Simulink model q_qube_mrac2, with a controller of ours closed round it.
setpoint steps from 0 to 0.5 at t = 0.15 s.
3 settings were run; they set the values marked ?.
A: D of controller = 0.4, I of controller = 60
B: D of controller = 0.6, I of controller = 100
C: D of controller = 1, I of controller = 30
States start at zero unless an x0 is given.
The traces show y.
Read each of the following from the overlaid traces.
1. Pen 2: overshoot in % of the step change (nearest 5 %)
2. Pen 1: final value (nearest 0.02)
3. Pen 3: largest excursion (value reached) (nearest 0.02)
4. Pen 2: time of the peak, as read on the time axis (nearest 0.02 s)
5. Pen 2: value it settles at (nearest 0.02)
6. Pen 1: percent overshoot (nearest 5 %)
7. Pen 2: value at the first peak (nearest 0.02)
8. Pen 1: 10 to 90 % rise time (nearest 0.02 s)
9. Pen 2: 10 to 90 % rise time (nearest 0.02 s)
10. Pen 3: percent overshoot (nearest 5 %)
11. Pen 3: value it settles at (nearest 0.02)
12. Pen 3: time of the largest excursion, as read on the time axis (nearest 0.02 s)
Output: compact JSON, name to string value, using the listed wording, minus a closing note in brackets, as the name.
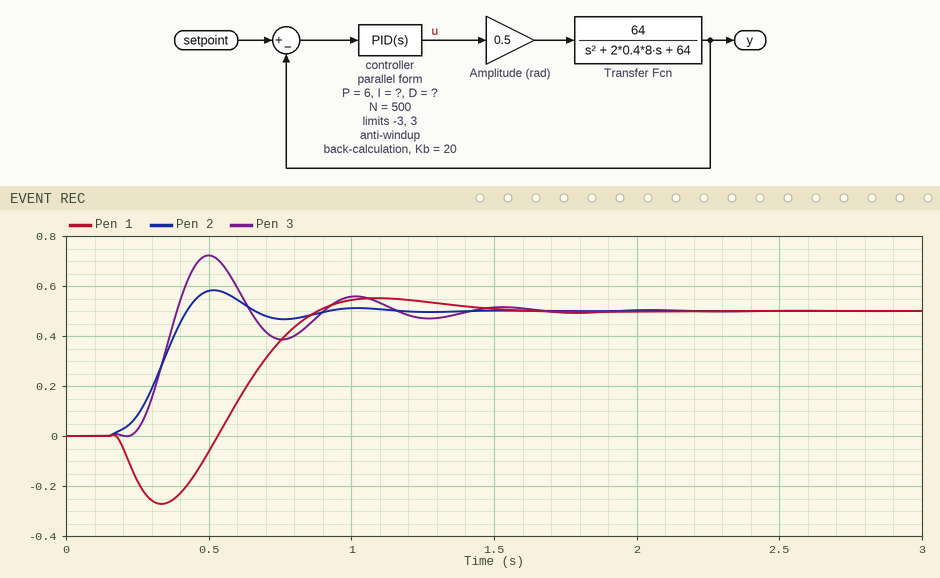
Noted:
{"Pen 2: overshoot in % of the step change": "15 %", "Pen 1: final value": "0.50", "Pen 3: largest excursion (value reached)": "0.72", "Pen 2: time of the peak, as read on the time axis": "0.52 s", "Pen 2: value it settles at": "0.50", "Pen 1: percent overshoot": "10 %", "Pen 2: value at the first peak": "0.58", "Pen 1: 10 to 90 % rise time": "0.26 s", "Pen 2: 10 to 90 % rise time": "0.18 s", "Pen 3: percent overshoot": "45 %", "Pen 3: value it settles at": "0.50", "Pen 3: time of the largest excursion, as read on the time axis": "0.50 s"}
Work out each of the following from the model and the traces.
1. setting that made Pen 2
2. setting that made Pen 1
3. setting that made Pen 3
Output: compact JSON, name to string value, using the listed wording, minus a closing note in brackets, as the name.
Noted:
{"setting that made Pen 2": "A", "setting that made Pen 1": "C", "setting that made Pen 3": "B"}
